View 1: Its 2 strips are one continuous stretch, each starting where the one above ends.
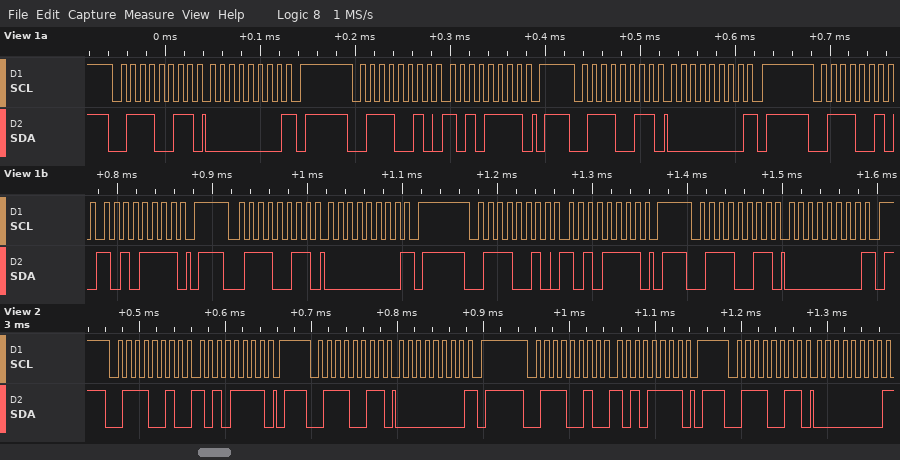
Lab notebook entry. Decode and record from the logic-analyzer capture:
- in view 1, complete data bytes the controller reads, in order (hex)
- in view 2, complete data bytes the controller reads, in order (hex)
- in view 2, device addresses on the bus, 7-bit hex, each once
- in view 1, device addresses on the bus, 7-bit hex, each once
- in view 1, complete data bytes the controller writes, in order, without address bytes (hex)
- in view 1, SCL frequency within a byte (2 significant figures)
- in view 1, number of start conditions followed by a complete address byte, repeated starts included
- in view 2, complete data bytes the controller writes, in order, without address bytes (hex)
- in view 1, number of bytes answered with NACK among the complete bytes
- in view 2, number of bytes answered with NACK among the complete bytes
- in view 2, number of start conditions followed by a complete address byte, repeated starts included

00 00 00 00
00 00
0x39
0x39
AF AF AF
100 kHz
7
AF AF
4
2
4
